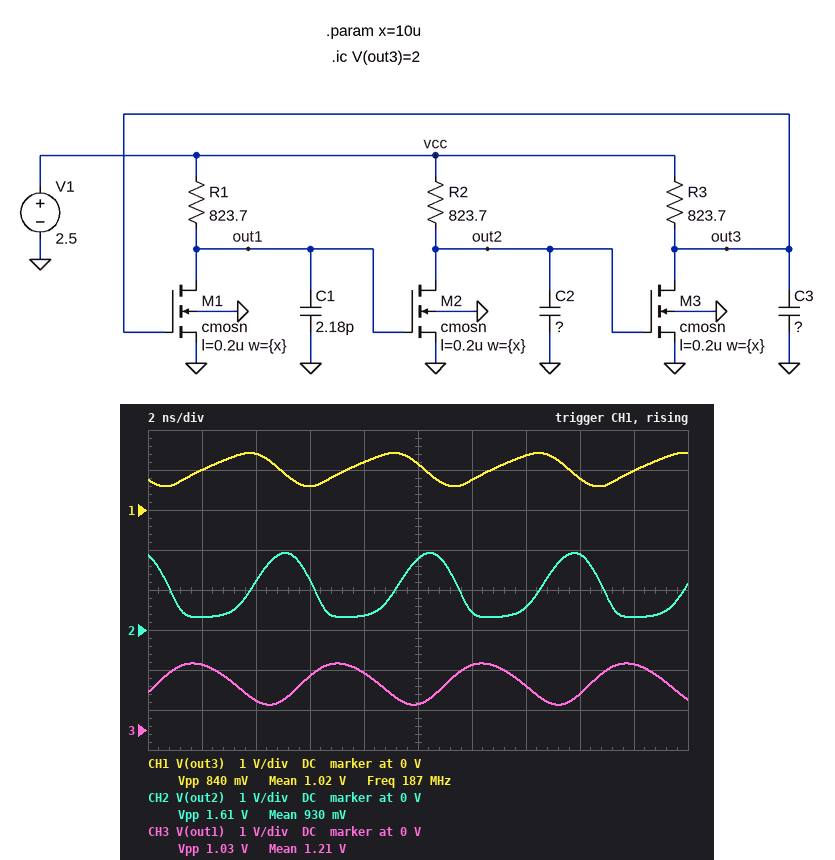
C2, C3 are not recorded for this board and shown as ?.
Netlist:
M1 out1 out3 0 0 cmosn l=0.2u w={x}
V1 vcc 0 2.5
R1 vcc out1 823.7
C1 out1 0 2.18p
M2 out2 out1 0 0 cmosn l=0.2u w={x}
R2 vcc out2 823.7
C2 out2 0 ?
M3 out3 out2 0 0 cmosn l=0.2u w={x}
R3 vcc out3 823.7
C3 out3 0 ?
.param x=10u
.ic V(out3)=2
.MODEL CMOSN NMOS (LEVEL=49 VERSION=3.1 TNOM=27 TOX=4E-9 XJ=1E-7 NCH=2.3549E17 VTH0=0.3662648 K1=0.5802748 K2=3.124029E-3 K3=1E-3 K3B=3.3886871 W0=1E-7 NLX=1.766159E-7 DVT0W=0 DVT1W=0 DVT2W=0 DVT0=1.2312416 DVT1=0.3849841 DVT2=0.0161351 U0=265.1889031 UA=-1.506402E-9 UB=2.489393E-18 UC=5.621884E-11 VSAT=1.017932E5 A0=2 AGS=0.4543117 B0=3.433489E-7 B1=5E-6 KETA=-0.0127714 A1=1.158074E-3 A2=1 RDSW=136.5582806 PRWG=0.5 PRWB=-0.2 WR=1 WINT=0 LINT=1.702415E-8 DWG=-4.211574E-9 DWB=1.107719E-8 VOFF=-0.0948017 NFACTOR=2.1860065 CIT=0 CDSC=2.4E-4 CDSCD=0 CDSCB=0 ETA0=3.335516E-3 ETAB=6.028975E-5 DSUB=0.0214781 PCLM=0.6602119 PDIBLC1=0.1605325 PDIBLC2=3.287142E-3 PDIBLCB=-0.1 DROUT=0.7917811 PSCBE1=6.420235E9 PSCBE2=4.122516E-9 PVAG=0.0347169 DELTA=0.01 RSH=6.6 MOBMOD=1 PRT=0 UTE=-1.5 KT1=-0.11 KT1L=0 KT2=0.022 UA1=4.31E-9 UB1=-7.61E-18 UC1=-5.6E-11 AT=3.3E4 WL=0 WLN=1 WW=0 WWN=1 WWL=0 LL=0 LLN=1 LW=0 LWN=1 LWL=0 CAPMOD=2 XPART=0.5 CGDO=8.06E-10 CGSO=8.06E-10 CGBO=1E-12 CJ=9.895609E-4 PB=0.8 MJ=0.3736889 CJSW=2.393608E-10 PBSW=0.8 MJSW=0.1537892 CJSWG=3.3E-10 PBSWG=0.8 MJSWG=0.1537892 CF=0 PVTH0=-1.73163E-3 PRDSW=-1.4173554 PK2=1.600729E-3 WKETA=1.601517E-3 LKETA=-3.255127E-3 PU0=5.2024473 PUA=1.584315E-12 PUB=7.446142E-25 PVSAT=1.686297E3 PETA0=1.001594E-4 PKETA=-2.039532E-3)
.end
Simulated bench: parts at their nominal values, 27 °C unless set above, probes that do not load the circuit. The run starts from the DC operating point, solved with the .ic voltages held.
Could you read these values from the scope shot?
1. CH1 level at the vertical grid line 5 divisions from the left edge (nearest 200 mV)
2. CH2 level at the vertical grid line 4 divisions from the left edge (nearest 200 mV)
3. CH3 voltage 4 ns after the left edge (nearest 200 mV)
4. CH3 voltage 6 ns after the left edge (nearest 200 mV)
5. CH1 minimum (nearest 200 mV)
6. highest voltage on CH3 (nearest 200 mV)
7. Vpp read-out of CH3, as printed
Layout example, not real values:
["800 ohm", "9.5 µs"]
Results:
["1.2 V", "400 mV", "800 mV", "1.4 V", "600 mV", "1.6 V", "1.03 V"]
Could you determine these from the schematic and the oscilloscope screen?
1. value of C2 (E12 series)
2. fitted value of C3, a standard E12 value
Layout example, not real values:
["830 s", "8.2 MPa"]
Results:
["1 pF", "5.6 pF"]
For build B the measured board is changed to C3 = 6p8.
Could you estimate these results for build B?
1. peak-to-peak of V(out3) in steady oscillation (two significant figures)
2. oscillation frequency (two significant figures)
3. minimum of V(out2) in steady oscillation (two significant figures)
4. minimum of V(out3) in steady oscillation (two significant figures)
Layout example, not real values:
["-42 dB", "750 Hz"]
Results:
["710 mV", "180 MHz", "330 mV", "670 mV"]
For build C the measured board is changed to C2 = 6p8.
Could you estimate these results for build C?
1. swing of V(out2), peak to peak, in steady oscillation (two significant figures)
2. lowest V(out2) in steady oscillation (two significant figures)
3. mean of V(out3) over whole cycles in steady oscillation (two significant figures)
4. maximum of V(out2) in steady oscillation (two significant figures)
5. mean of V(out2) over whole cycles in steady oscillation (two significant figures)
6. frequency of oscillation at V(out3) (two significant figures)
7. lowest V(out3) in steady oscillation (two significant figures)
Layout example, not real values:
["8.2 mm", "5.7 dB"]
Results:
["1.2 V", "390 mV", "1.1 V", "1.6 V", "1.0 V", "99 MHz", "560 mV"]
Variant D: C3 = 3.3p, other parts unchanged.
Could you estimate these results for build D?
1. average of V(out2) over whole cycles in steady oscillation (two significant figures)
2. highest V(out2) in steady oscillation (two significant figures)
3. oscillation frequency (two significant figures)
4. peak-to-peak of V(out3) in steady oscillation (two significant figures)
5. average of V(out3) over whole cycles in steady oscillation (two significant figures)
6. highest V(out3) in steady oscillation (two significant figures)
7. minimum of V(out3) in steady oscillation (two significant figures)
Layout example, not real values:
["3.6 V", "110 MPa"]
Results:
["1.0 V", "2.0 V", "220 MHz", "1.1 V", "1.0 V", "1.6 V", "420 mV"]
